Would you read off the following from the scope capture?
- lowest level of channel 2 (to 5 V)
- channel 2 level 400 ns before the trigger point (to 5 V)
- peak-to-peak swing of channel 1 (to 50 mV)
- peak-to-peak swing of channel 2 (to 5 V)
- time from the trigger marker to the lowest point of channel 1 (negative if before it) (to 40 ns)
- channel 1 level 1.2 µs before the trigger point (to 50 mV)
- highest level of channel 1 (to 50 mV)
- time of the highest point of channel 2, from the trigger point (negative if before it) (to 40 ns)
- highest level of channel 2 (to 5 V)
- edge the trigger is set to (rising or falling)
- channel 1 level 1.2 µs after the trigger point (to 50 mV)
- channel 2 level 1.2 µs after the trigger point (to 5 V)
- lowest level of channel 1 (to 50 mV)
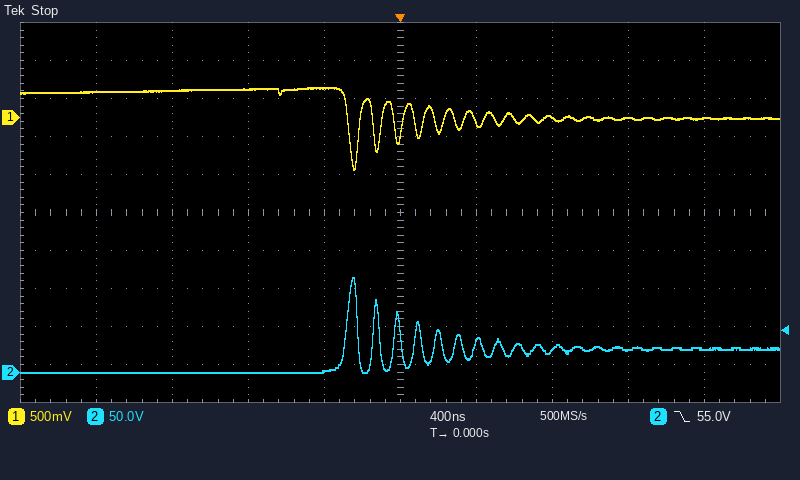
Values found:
0 V
0 V
1.10 V
125 V
-240 ns
350 mV
400 mV
-240 ns
125 V
falling
0 mV
30 V
-700 mV
